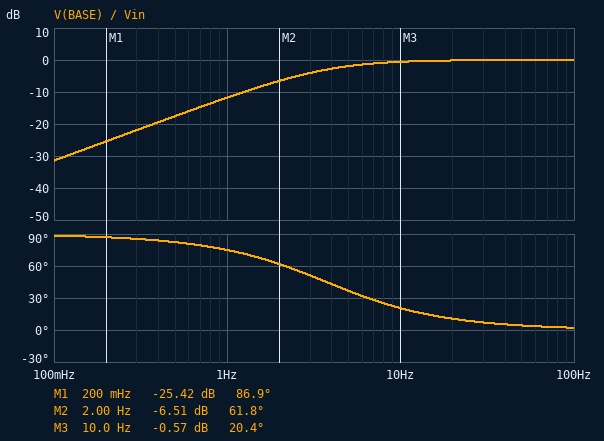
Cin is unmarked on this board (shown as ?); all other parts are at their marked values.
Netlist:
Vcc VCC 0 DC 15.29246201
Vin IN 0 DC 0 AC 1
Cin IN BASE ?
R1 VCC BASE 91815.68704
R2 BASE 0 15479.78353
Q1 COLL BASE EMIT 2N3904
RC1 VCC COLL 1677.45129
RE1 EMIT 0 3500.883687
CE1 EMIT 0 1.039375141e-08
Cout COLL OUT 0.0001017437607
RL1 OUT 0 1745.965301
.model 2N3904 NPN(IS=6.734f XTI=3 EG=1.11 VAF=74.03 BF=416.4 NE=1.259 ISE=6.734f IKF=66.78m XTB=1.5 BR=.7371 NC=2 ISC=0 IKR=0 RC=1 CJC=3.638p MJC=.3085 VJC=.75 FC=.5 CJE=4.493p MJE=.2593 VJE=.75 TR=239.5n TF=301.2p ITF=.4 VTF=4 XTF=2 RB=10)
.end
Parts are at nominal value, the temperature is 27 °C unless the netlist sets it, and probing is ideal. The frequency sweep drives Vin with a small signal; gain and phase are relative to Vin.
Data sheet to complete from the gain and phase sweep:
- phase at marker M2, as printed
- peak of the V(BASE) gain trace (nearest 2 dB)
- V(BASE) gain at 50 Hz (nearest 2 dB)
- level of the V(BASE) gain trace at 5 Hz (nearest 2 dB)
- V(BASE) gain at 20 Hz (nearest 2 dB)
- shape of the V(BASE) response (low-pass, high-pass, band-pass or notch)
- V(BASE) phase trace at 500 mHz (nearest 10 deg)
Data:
61.8 deg
0 dB
0 dB
-2 dB
0 dB
high-pass
80 deg
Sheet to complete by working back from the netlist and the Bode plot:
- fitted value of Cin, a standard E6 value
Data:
3.3 µF
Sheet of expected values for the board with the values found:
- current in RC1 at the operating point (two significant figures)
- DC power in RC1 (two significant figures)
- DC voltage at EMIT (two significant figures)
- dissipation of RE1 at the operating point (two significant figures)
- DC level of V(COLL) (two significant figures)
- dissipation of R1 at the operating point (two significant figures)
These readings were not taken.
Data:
430 µA
310 µW
1.5 V
660 µW
15 V
1.9 mW
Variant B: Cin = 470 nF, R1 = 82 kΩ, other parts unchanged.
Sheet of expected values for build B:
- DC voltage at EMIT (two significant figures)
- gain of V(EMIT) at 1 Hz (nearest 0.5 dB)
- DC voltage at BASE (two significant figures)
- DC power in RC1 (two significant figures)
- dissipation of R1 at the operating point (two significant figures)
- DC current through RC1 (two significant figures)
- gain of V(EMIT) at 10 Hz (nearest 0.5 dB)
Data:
1.7 V
-28.5 dB
2.4 V
410 µW
2.0 mW
490 µA
-9.0 dB
